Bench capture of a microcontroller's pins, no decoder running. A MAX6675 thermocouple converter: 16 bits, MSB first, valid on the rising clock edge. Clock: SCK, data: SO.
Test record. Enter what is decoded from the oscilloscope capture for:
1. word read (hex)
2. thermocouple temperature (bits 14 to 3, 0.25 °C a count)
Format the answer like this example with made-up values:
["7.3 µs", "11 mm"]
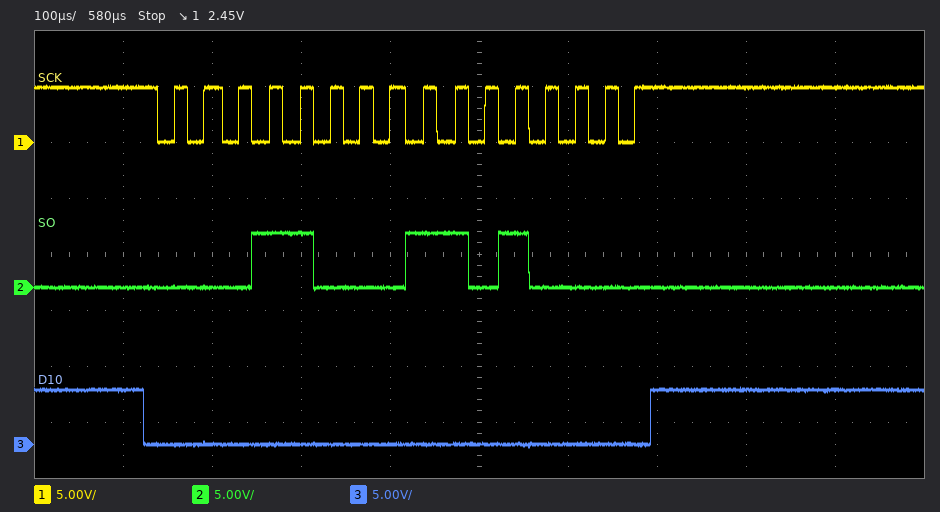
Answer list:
["0x18D0", "198.50 °C"]
